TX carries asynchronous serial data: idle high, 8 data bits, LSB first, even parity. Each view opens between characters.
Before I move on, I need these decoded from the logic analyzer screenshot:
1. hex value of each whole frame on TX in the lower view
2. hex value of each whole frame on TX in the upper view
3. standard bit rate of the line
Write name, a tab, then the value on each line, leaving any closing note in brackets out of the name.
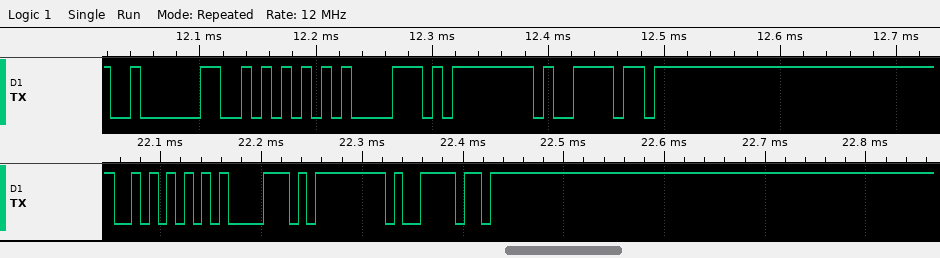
hex value of each whole frame on TX in the lower view	AA, E1, FF, DE
hex value of each whole frame on TX in the upper view	02, AA, E1, FF, DE
standard bit rate of the line	115200 baud
